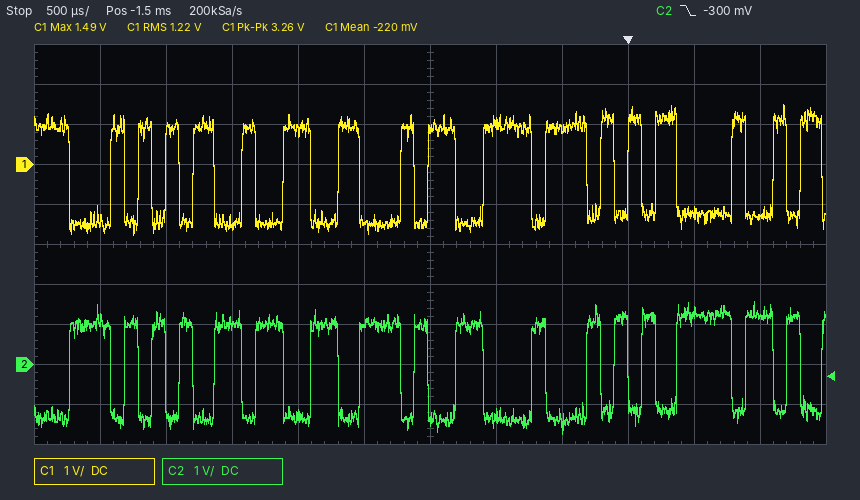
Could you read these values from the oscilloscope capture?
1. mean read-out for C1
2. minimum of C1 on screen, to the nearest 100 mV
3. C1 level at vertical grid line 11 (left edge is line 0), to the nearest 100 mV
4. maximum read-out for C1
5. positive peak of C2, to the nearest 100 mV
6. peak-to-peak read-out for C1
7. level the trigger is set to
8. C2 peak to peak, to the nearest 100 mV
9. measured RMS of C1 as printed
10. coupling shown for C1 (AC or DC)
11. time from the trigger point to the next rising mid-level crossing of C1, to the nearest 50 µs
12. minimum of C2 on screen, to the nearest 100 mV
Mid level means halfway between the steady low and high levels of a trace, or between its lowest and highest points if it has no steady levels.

-220 mV
-1.8 V
-1.3 V
1.49 V
1.6 V
3.26 V
-300 mV
3.3 V
1.22 V
DC
200 µs
-1.7 V
